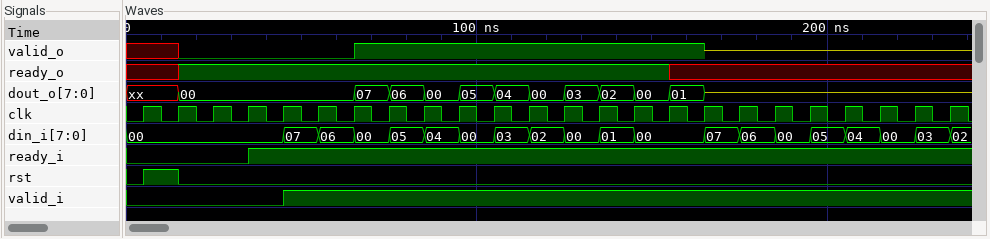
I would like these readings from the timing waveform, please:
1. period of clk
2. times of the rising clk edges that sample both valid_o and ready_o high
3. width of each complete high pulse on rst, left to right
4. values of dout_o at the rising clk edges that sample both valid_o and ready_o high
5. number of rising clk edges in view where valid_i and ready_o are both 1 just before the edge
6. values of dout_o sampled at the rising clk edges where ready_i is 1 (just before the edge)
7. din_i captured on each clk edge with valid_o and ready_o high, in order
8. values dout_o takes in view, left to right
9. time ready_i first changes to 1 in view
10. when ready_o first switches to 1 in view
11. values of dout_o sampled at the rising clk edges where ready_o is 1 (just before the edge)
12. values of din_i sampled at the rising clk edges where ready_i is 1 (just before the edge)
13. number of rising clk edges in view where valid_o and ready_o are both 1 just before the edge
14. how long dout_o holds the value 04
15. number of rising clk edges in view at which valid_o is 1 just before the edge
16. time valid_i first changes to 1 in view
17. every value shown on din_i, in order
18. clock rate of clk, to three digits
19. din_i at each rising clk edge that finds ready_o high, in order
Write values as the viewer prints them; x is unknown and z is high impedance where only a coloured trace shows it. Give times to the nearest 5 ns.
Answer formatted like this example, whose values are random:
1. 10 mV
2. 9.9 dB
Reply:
1. 10 ns
2. 75 ns, 85 ns, 95 ns, 105 ns, 115 ns, 125 ns, 135 ns, 145 ns, 155 ns
3. 10 ns
4. 07, 06, 00, 05, 04, 00, 03, 02, 00
5. 11
6. 00, 00, 00, 07, 06, 00, 05, 04, 00, 03, 02, 00, 01, z, z, z, z, z, z, z
7. 00, 05, 04, 00, 03, 02, 00, 01, 00
8. xx, 00, 07, 06, 00, 05, 04, 00, 03, 02, 00, 01, z
9. 35 ns
10. 15 ns
11. 00, 00, 00, 00, 00, 07, 06, 00, 05, 04, 00, 03, 02, 00
12. 00, 07, 06, 00, 05, 04, 00, 03, 02, 00, 01, 00, 00, 07, 06, 00, 05, 04, 00, 03
13. 9
14. 10 ns
15. 10
16. 45 ns
17. 00, 07, 06, 00, 05, 04, 00, 03, 02, 00, 01, 00, 07, 06, 00, 05, 04, 00, 03, 02
18. 100 MHz
19. 00, 00, 00, 07, 06, 00, 05, 04, 00, 03, 02, 00, 01, 00
